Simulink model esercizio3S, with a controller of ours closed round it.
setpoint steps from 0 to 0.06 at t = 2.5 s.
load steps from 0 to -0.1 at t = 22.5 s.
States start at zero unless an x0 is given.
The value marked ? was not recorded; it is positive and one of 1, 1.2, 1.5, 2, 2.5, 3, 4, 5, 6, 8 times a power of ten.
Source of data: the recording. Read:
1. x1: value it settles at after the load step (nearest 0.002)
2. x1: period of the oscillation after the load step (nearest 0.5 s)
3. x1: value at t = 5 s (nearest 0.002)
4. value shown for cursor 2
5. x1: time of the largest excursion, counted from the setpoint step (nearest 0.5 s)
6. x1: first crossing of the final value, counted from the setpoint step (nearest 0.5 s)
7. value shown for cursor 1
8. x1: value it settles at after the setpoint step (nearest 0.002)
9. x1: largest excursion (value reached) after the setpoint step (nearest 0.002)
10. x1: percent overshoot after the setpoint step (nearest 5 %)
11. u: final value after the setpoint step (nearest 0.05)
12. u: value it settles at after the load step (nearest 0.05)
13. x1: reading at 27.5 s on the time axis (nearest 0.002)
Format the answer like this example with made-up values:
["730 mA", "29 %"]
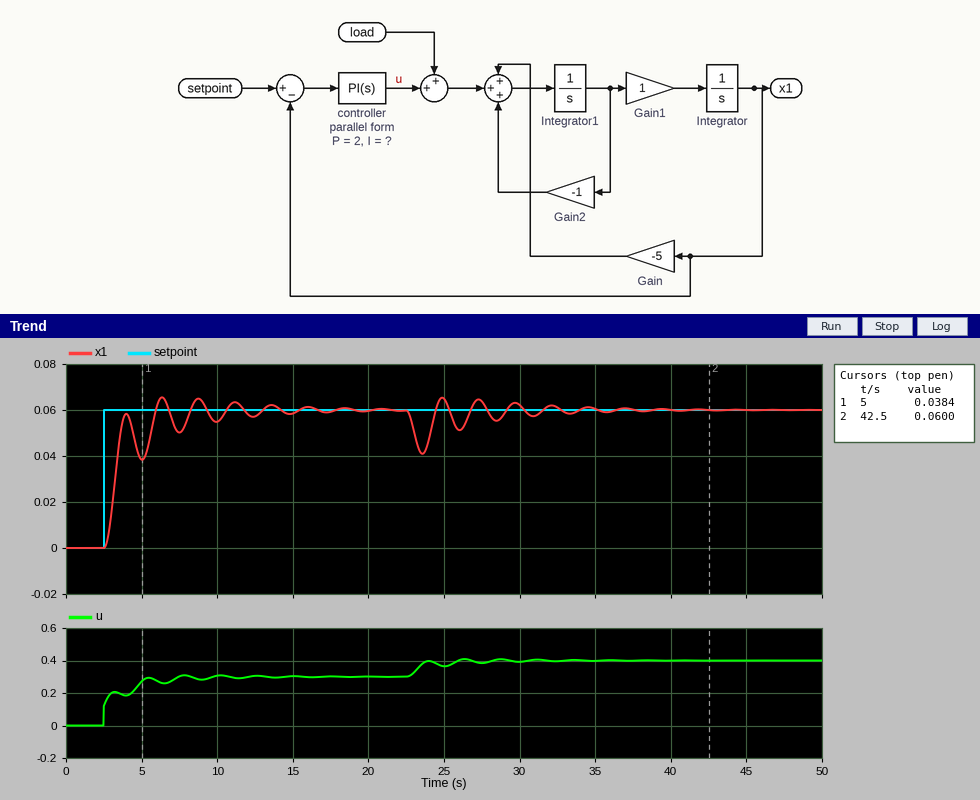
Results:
["0.060", "2.5 s", "0.038", "0.0600", "4.0 s", "3.5 s", "0.0384", "0.060", "0.066", "10 %", "0.30", "0.40", "0.064"]
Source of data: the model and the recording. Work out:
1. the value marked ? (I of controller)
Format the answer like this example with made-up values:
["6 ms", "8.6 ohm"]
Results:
["4"]
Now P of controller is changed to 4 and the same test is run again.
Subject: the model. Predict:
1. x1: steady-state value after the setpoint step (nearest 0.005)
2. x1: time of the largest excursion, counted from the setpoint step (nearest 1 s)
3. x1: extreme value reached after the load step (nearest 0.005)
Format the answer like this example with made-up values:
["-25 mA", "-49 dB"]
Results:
["0.060", "3 s", "0.045"]
